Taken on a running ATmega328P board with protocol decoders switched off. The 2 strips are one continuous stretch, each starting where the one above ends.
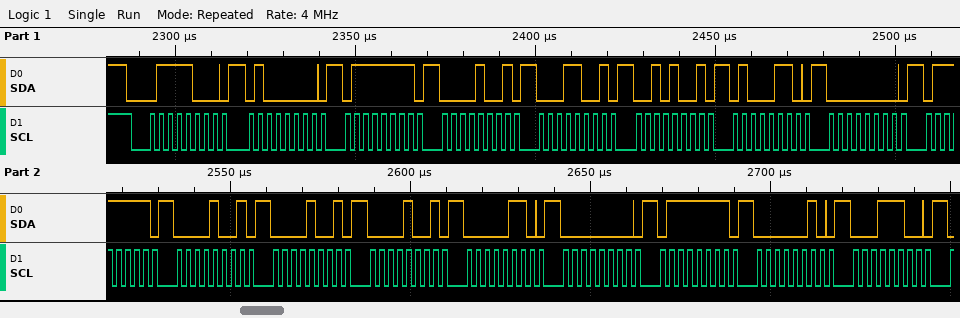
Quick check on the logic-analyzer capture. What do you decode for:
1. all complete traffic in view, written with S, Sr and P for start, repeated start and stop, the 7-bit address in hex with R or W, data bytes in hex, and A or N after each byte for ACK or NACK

S 3CW A 40 A 7F A 09 A 19 A 29 A 46 A 00 A 7F A 09 A 09 A 09 A 06 A 00 A 7F A 02 A 1C A
